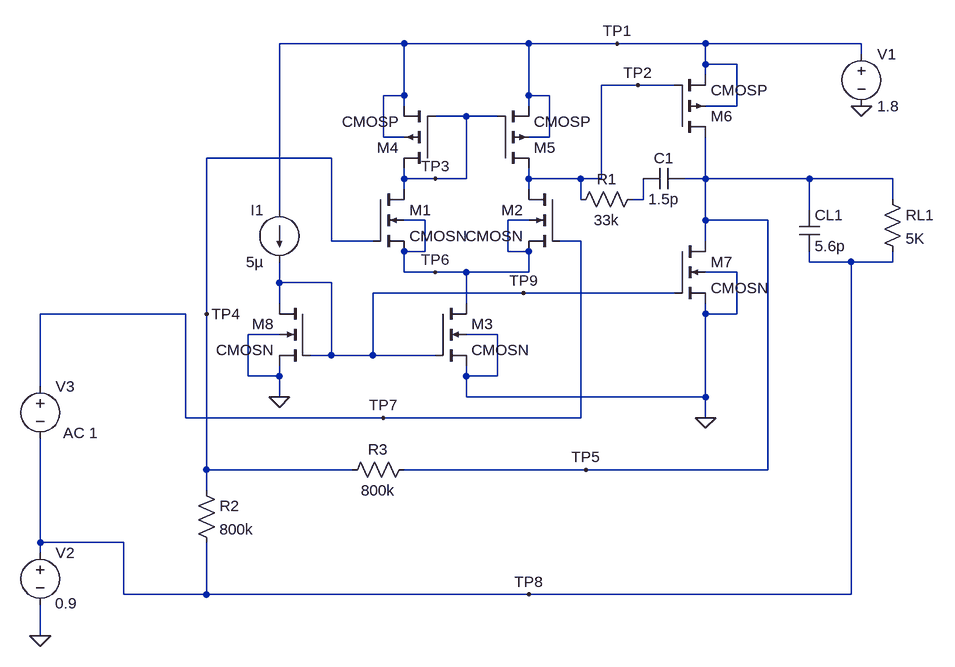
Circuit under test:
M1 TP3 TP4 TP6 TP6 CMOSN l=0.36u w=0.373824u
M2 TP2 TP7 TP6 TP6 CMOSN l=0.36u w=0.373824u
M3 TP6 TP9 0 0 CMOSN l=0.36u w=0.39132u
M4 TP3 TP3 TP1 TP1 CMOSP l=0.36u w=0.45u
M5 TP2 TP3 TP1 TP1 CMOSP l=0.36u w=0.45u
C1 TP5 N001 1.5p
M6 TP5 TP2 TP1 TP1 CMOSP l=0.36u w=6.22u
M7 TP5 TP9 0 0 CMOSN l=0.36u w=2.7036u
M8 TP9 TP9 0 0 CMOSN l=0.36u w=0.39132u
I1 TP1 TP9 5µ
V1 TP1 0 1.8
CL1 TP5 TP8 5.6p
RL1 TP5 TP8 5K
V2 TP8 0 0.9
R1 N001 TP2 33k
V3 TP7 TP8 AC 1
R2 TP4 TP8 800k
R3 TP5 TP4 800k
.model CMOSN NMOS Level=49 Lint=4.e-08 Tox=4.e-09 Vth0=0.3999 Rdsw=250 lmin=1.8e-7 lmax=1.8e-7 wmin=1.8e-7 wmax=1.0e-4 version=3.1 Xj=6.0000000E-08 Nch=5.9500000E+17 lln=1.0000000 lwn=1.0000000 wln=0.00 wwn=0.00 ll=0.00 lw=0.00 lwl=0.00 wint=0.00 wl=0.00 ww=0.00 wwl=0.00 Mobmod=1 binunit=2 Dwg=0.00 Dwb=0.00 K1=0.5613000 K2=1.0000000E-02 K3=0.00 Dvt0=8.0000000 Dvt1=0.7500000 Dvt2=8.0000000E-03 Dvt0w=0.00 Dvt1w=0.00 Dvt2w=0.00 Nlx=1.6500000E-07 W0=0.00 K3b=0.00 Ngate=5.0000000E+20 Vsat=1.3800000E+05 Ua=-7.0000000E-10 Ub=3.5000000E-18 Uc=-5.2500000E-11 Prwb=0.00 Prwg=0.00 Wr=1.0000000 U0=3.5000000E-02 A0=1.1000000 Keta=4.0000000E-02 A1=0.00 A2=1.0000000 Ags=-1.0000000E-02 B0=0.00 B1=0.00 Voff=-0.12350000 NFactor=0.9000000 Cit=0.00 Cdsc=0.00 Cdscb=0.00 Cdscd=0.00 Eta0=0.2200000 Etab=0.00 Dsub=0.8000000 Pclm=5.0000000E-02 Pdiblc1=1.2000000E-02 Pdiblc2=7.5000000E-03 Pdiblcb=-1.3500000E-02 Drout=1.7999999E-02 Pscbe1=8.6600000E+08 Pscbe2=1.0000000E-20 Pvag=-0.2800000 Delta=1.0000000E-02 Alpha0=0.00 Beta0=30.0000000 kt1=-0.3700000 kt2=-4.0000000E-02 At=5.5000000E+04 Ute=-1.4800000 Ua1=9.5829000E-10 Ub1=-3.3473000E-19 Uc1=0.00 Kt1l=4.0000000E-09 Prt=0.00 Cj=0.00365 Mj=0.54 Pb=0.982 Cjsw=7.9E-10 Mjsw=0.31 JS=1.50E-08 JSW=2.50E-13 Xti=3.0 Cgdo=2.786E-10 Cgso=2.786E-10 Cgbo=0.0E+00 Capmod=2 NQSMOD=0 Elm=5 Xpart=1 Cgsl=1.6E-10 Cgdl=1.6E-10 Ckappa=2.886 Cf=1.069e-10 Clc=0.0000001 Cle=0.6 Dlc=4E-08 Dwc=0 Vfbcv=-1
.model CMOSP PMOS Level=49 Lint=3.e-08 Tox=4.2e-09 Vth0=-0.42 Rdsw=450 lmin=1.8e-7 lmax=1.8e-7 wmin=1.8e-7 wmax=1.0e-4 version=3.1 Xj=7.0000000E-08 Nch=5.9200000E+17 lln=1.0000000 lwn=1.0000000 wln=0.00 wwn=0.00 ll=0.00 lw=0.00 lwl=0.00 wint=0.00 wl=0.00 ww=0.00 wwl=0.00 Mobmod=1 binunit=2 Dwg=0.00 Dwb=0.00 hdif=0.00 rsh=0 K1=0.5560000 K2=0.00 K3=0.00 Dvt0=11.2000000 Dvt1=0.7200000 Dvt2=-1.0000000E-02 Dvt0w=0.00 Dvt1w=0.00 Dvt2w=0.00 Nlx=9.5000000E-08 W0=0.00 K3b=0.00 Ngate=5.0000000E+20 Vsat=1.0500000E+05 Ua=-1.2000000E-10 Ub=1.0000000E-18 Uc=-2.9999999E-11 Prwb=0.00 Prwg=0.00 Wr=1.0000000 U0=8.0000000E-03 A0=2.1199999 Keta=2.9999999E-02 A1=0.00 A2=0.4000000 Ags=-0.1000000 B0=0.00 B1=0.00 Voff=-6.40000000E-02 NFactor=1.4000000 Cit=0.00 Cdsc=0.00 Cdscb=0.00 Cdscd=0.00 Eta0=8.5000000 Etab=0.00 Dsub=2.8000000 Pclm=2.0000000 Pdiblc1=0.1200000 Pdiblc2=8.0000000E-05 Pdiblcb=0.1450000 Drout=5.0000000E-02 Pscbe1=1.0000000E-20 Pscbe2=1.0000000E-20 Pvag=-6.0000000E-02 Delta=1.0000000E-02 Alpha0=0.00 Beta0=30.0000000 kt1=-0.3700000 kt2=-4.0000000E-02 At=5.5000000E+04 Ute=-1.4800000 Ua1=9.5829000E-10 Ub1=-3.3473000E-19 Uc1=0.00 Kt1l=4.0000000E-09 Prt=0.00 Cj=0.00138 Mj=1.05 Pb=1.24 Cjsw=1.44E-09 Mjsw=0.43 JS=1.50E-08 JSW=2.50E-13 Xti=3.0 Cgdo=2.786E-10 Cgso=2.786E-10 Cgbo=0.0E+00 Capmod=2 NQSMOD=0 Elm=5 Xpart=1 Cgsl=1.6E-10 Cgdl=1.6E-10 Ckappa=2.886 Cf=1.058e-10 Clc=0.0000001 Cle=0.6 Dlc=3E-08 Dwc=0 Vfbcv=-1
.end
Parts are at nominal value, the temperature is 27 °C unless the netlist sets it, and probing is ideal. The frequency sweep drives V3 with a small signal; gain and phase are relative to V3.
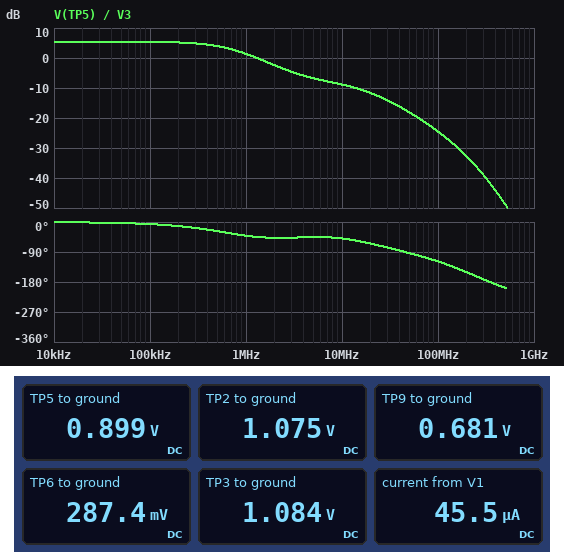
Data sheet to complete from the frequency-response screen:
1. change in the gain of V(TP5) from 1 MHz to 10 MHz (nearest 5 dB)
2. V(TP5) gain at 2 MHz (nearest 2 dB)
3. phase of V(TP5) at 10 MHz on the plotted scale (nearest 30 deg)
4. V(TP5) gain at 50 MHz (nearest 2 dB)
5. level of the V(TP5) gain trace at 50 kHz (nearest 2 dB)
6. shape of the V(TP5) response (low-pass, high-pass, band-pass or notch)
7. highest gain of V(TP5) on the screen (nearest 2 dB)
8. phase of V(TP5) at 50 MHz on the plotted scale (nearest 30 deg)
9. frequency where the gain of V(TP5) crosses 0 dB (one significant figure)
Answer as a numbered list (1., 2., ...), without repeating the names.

1. -10 dB
2. -2 dB
3. -60 deg
4. -18 dB
5. 6 dB
6. low-pass
7. 6 dB
8. -90 deg
9. 1 MHz
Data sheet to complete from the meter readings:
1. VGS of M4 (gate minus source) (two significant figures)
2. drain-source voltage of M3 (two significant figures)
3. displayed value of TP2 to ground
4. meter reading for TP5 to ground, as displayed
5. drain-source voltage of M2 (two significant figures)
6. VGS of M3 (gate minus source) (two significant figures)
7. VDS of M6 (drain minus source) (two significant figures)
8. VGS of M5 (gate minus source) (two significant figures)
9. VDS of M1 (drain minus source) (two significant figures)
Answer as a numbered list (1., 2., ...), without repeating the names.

1. -720 mV
2. 290 mV
3. 1.075 V
4. 0.899 V
5. 790 mV
6. 680 mV
7. -900 mV
8. -720 mV
9. 800 mV
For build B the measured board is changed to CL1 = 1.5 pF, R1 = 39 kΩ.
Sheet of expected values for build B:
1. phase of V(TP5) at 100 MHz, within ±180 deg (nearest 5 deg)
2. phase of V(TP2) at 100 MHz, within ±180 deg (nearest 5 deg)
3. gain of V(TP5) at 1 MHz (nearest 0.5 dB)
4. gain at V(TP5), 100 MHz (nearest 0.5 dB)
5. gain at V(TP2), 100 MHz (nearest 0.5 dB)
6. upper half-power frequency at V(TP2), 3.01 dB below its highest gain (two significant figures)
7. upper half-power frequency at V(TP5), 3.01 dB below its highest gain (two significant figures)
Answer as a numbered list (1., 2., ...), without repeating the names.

1. -95 deg
2. 160 deg
3. 1.0 dB
4. -12.0 dB
5. -0.5 dB
6. 780 kHz
7. 750 kHz
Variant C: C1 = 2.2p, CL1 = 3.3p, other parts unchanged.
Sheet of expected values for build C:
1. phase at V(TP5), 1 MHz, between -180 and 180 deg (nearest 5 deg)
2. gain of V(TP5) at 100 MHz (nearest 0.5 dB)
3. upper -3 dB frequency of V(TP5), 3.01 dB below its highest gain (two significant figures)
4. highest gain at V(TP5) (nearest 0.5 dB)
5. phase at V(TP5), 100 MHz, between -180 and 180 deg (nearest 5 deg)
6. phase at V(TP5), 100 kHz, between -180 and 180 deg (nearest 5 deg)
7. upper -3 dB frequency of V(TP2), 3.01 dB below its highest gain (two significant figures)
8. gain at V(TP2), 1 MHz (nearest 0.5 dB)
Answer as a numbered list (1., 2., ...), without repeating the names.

1. -45 deg
2. -20.0 dB
3. 530 kHz
4. 5.5 dB
5. -110 deg
6. -10 deg
7. 550 kHz
8. -2.5 dB
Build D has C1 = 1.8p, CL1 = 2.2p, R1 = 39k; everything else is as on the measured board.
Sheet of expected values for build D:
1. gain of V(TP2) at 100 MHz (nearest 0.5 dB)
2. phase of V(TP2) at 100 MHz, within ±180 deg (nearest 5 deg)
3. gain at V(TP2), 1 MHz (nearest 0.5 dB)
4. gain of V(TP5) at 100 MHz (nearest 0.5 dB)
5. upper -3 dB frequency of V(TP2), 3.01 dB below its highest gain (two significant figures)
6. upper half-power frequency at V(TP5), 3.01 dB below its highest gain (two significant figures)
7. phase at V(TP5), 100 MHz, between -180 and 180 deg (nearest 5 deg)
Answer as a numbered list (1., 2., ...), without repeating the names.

1. 0 dB
2. 155 deg
3. -1.5 dB
4. -15.0 dB
5. 650 kHz
6. 630 kHz
7. -105 deg
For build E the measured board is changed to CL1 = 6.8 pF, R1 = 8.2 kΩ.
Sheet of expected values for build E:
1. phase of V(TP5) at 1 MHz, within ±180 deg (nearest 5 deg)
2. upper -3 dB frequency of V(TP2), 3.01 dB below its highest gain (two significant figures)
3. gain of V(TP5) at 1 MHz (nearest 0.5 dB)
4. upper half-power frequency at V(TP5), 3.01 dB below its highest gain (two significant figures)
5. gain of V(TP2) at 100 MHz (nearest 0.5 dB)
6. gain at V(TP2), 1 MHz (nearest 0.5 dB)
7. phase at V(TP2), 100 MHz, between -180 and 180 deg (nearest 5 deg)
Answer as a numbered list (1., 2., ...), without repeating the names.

1. -50 deg
2. 1.0 MHz
3. 2.0 dB
4. 940 kHz
5. -13.0 dB
6. 0 dB
7. 155 deg
